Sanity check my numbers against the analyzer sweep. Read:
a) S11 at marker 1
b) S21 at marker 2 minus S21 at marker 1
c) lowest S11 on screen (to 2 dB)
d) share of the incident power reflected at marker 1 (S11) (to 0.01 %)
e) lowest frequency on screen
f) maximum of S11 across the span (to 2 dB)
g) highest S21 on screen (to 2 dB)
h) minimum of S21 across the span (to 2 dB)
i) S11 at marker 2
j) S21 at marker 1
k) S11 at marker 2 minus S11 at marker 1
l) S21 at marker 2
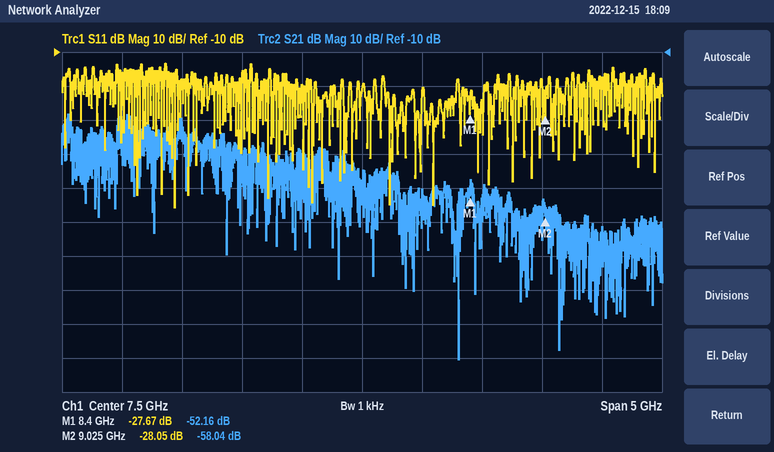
-27.67 dB
-5.88 dB
-56 dB
0.17 %
5 GHz
-14 dB
-28 dB
-100 dB
-28.05 dB
-52.16 dB
-0.38 dB
-58.04 dB
